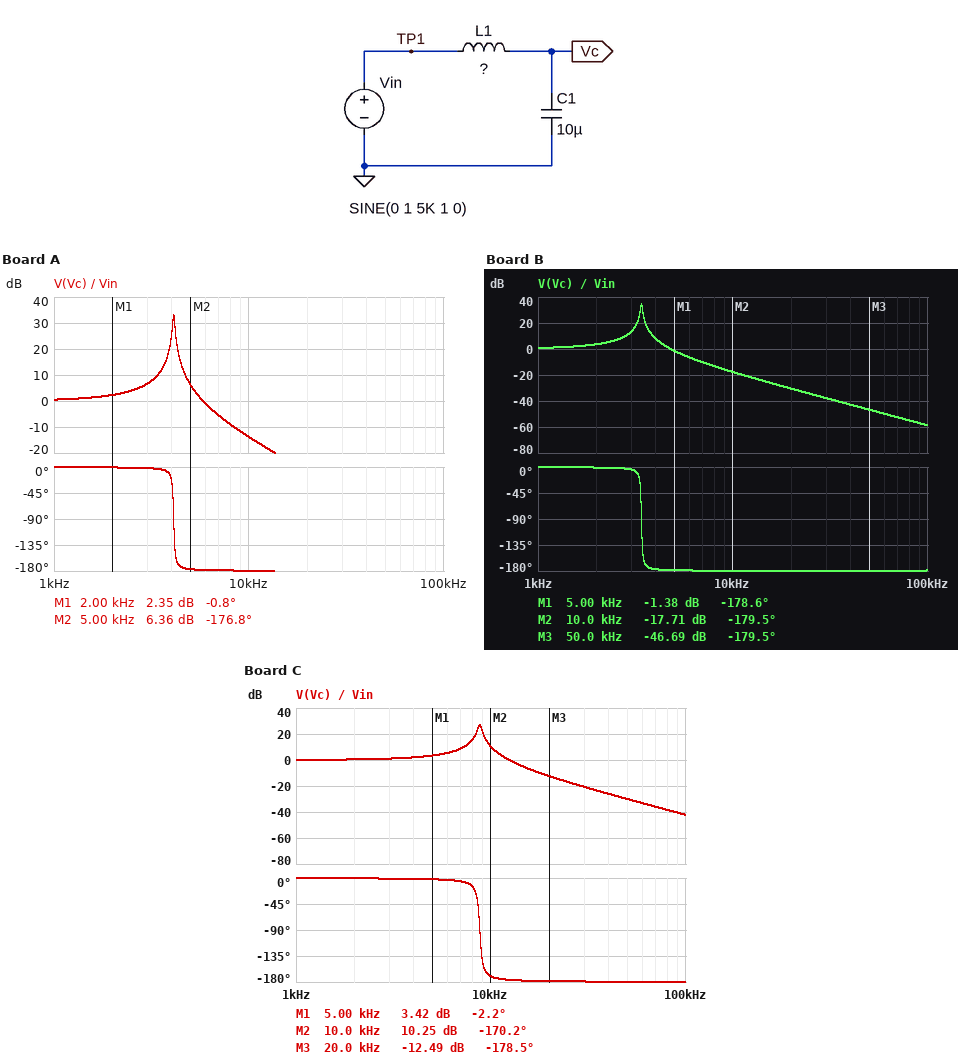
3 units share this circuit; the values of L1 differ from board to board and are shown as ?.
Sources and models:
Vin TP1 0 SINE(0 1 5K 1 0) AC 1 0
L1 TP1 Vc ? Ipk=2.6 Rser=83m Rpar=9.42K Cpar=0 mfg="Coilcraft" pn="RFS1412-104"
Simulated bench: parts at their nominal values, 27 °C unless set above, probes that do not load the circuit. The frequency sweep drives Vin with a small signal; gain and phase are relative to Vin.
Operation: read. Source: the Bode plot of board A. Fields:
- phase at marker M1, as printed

-0.8 deg
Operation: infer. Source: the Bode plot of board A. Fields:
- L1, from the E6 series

150 µH
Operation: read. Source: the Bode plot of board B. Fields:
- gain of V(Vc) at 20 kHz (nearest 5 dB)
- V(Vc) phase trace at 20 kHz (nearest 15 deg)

-30 dB
-180 deg
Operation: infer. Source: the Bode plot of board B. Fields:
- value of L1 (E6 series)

220 µH
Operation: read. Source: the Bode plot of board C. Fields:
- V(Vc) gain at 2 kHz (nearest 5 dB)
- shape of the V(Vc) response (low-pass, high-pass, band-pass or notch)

0 dB
low-pass
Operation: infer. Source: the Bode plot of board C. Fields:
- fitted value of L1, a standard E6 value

33 µH
